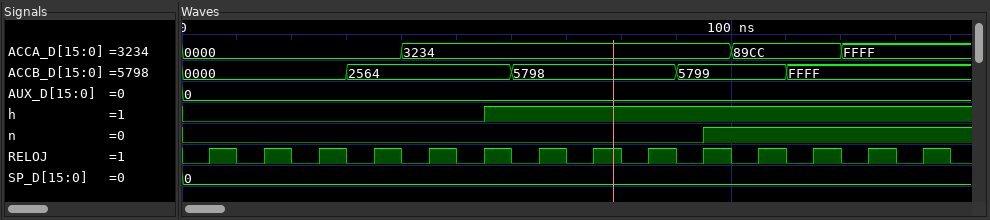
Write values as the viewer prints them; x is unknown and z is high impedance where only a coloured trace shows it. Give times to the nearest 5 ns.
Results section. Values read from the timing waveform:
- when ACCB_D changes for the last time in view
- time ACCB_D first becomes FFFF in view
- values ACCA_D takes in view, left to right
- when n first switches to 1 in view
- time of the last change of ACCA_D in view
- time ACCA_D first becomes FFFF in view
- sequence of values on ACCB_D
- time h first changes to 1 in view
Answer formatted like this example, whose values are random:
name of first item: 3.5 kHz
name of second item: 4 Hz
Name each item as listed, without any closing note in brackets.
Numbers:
when ACCB_D changes for the last time in view: 110 ns
time ACCB_D first becomes FFFF in view: 110 ns
values ACCA_D takes in view, left to right: 0000, 3234, 89CC, FFFF
when n first switches to 1 in view: 95 ns
time of the last change of ACCA_D in view: 120 ns
time ACCA_D first becomes FFFF in view: 120 ns
sequence of values on ACCB_D: 0000, 2564, 5798, 5799, FFFF
time h first changes to 1 in view: 55 ns
